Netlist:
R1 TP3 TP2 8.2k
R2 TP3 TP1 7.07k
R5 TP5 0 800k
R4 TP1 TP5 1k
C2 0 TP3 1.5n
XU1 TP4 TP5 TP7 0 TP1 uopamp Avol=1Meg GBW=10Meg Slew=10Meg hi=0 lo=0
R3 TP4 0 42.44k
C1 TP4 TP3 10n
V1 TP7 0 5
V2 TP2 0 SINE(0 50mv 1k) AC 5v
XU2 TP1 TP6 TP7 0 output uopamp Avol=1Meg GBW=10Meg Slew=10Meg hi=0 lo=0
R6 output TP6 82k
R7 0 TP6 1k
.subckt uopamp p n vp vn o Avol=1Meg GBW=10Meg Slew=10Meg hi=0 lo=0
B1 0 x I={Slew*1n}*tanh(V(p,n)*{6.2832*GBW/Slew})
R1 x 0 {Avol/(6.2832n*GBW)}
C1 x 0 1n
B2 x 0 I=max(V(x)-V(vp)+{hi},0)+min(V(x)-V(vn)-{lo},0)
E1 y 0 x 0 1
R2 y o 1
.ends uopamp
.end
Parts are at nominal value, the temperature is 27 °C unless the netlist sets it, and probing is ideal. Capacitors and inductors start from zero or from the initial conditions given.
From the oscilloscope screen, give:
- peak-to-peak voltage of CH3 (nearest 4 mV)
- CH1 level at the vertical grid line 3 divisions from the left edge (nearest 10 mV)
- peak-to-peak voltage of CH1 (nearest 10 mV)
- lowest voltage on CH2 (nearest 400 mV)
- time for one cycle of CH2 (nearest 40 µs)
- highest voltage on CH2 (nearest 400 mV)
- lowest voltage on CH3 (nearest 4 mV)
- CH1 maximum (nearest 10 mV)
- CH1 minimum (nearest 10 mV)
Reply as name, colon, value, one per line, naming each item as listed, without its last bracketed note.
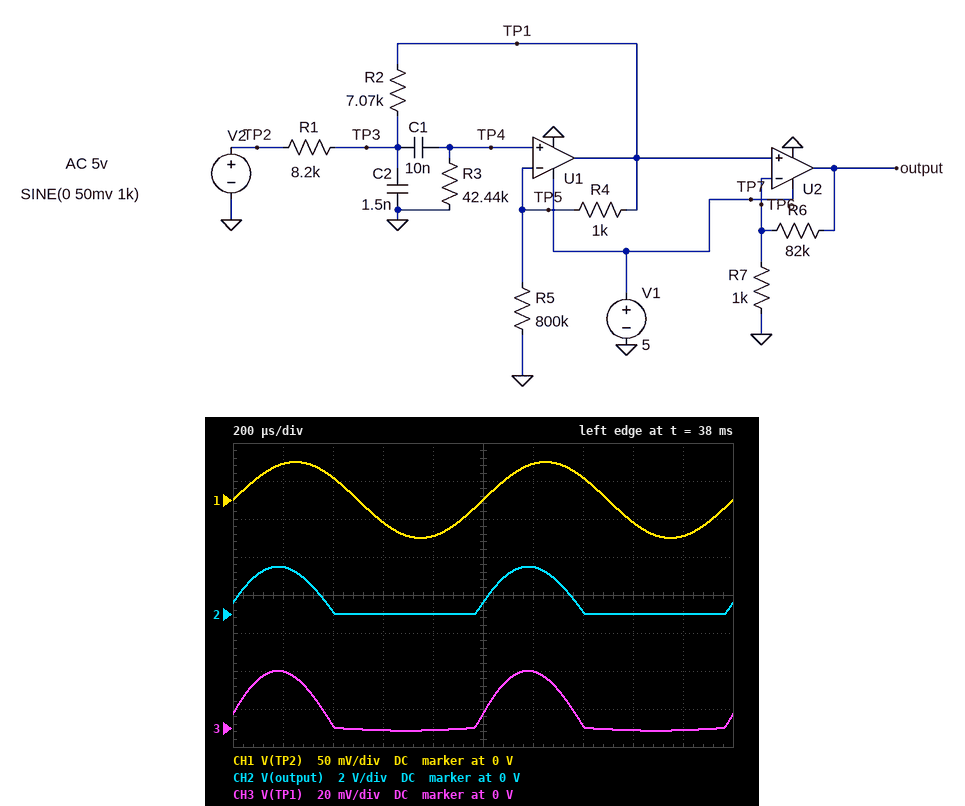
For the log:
peak-to-peak voltage of CH3: 32 mV
CH1 level at the vertical grid line 3 divisions from the left edge: -30 mV
peak-to-peak voltage of CH1: 100 mV
lowest voltage on CH2: 0 V
time for one cycle of CH2: 1.00 ms
highest voltage on CH2: 2.4 V
lowest voltage on CH3: 0 V
CH1 maximum: 50 mV
CH1 minimum: -50 mV
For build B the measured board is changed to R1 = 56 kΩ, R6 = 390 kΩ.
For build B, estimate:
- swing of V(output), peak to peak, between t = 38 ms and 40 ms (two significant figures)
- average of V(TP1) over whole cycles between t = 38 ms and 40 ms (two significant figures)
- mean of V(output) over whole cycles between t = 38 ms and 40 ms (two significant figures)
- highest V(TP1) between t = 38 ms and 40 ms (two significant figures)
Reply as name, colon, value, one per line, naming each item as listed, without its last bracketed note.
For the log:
swing of V(output), peak to peak, between t = 38 ms and 40 ms: 4.1 V
average of V(TP1) over whole cycles between t = 38 ms and 40 ms: 2.3 mV
mean of V(output) over whole cycles between t = 38 ms and 40 ms: 970 mV
highest V(TP1) between t = 38 ms and 40 ms: 11 mV
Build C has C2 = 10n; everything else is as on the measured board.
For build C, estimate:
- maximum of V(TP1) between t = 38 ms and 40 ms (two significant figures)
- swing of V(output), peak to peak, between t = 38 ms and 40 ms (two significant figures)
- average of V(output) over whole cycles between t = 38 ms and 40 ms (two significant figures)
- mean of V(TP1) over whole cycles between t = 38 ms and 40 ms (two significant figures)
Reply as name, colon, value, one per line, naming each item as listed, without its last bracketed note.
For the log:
maximum of V(TP1) between t = 38 ms and 40 ms: 29 mV
swing of V(output), peak to peak, between t = 38 ms and 40 ms: 2.4 V
average of V(output) over whole cycles between t = 38 ms and 40 ms: 690 mV
mean of V(TP1) over whole cycles between t = 38 ms and 40 ms: 7.8 mV
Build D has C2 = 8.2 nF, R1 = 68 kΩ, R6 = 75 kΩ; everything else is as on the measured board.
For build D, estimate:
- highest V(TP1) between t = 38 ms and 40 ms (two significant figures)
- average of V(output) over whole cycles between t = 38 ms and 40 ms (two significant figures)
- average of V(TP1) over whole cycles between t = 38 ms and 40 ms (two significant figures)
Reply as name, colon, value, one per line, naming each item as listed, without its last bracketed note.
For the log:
highest V(TP1) between t = 38 ms and 40 ms: 7.3 mV
average of V(output) over whole cycles between t = 38 ms and 40 ms: 150 mV
average of V(TP1) over whole cycles between t = 38 ms and 40 ms: 1.9 mV
